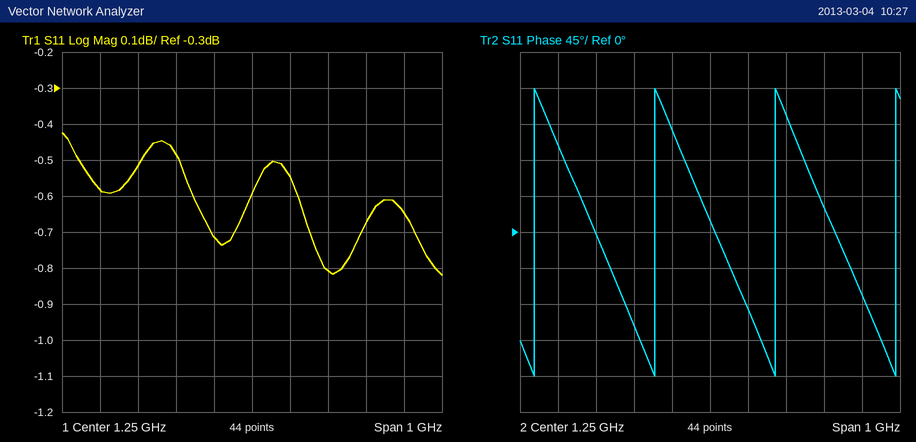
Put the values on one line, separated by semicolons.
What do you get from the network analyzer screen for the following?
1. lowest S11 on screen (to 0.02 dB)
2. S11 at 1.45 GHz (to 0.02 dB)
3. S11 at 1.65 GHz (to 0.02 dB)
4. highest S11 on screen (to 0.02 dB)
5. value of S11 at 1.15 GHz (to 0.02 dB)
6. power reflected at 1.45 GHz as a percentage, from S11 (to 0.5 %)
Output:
-0.82 dB; -0.80 dB; -0.64 dB; -0.42 dB; -0.72 dB; 83.0 %
